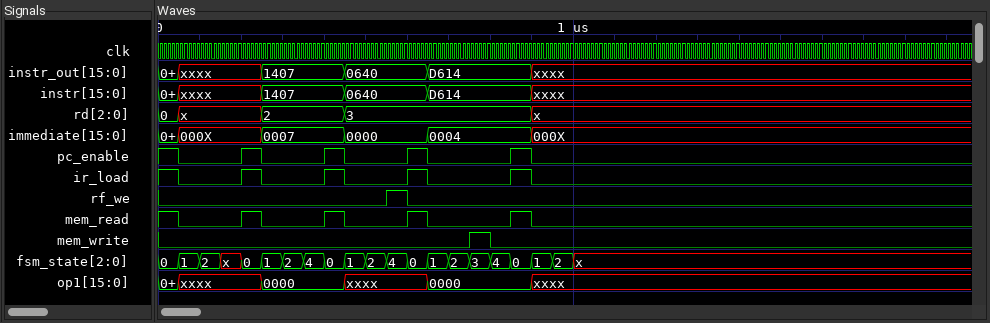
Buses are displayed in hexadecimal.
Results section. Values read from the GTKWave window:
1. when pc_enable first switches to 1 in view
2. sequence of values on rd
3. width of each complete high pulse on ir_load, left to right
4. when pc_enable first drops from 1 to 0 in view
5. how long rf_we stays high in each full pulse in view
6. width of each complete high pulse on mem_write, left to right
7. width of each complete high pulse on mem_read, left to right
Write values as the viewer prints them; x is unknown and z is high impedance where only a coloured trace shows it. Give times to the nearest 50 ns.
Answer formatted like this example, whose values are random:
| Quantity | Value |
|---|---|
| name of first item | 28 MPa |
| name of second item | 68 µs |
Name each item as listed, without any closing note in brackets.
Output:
| Quantity | Value |
|---|---|
| when pc_enable first switches to 1 in view | 200 ns |
| sequence of values on rd | 0, x, 2, 3, x |
| width of each complete high pulse on ir_load, left to right | 50 ns, 50 ns, 50 ns, 50 ns |
| when pc_enable first drops from 1 to 0 in view | 50 ns |
| how long rf_we stays high in each full pulse in view | 50 ns |
| width of each complete high pulse on mem_write, left to right | 50 ns |
| width of each complete high pulse on mem_read, left to right | 50 ns, 50 ns, 50 ns, 50 ns |
